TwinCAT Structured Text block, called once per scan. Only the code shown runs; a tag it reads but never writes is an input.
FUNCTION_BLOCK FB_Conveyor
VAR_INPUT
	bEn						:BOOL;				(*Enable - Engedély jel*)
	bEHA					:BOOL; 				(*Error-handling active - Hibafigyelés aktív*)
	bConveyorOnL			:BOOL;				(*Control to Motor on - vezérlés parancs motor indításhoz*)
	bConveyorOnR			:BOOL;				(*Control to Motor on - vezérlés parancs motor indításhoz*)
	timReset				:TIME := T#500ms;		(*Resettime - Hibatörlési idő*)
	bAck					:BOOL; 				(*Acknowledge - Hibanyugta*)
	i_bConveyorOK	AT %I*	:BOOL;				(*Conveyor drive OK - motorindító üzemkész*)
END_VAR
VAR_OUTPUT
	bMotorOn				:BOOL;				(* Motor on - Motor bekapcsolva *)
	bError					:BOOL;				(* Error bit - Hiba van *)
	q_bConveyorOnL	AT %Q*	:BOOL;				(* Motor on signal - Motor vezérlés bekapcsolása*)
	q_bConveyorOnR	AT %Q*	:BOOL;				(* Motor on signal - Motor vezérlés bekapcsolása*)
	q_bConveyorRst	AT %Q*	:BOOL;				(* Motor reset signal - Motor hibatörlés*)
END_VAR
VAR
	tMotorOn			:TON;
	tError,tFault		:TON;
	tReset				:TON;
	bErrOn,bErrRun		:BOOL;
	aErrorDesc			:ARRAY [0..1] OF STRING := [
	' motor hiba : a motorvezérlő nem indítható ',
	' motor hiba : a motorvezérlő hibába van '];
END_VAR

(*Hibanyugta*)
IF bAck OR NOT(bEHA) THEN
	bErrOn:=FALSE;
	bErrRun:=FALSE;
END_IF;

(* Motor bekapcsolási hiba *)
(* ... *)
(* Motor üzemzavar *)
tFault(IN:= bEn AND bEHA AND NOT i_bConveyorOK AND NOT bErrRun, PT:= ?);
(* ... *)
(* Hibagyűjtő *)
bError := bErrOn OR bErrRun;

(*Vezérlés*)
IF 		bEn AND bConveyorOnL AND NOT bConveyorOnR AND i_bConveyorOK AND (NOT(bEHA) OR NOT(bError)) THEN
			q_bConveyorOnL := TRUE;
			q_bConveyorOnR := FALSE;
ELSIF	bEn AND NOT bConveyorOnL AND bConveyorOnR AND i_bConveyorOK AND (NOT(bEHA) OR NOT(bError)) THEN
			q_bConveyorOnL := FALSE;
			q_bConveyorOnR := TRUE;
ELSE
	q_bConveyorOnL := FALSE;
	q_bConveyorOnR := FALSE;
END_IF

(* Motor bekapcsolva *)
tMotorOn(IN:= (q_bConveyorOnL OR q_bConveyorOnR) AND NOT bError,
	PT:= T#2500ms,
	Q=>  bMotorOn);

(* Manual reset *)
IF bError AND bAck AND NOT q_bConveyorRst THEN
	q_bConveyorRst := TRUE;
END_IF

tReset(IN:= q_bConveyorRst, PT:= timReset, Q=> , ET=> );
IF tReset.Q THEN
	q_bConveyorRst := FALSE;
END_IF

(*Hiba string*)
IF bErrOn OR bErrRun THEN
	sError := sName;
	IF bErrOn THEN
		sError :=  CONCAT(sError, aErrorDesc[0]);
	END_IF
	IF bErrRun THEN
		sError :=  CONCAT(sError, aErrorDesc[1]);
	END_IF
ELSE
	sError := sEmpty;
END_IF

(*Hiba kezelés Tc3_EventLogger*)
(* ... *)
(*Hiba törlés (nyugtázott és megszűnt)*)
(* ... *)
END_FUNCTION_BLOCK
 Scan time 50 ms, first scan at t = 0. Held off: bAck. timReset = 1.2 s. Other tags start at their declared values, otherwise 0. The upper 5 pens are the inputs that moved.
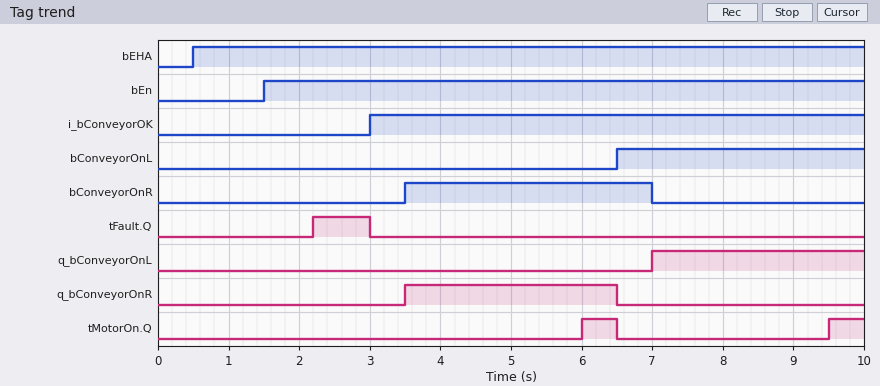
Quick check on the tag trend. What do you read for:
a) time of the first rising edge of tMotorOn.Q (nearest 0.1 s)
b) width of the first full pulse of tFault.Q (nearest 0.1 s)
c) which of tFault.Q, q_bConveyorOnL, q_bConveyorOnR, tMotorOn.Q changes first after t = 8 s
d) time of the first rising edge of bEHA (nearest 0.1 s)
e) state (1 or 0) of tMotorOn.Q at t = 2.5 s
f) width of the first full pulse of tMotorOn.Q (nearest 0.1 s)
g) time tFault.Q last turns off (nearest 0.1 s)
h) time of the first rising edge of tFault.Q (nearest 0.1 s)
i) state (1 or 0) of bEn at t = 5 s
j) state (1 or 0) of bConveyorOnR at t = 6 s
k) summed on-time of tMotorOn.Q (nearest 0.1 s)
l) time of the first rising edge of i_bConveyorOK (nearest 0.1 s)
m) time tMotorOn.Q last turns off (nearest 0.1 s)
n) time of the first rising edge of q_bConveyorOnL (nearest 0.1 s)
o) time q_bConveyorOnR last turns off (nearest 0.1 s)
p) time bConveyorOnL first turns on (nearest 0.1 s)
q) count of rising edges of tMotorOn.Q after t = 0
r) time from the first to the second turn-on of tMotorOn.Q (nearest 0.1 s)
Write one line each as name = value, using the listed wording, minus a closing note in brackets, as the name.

time of the first rising edge of tMotorOn.Q = 6.0 s
width of the first full pulse of tFault.Q = 0.8 s
which of tFault.Q, q_bConveyorOnL, q_bConveyorOnR, tMotorOn.Q changes first after t = 8 s = tMotorOn.Q
time of the first rising edge of bEHA = 0.5 s
state (1 or 0) of tMotorOn.Q at t = 2.5 s = 0
width of the first full pulse of tMotorOn.Q = 0.5 s
time tFault.Q last turns off = 3.0 s
time of the first rising edge of tFault.Q = 2.2 s
state (1 or 0) of bEn at t = 5 s = 1
state (1 or 0) of bConveyorOnR at t = 6 s = 1
summed on-time of tMotorOn.Q = 1.0 s
time of the first rising edge of i_bConveyorOK = 3.0 s
time tMotorOn.Q last turns off = 6.5 s
time of the first rising edge of q_bConveyorOnL = 7.0 s
time q_bConveyorOnR last turns off = 6.5 s
time bConveyorOnL first turns on = 6.5 s
count of rising edges of tMotorOn.Q after t = 0 = 2
time from the first to the second turn-on of tMotorOn.Q = 3.5 s
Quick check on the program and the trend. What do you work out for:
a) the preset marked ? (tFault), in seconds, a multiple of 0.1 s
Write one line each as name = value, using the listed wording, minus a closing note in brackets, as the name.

the preset marked ? (tFault), in seconds, a multiple of 0.1 s = 0.7 s
